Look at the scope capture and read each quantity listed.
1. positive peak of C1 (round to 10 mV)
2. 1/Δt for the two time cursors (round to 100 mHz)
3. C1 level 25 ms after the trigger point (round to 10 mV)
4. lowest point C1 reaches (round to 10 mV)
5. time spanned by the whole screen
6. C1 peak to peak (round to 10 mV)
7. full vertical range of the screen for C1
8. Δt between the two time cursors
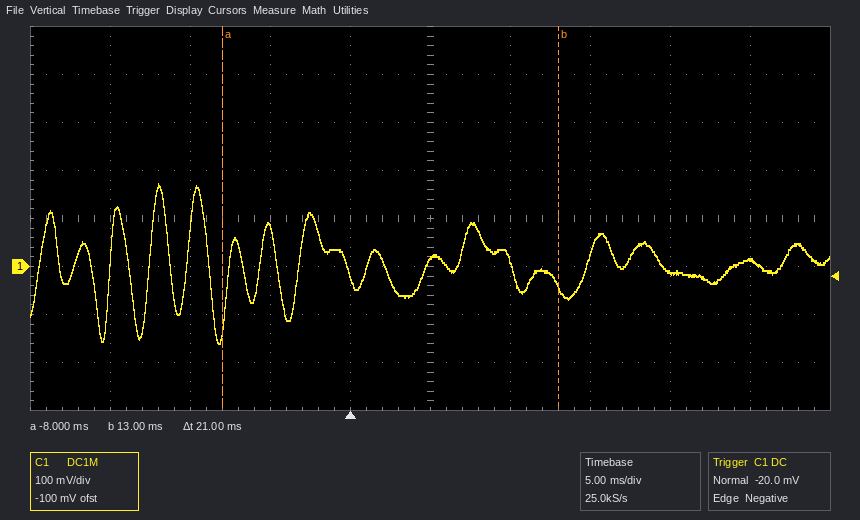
170 mV
47.6 Hz
10 mV
-160 mV
50 ms
330 mV
800 mV
21 ms
